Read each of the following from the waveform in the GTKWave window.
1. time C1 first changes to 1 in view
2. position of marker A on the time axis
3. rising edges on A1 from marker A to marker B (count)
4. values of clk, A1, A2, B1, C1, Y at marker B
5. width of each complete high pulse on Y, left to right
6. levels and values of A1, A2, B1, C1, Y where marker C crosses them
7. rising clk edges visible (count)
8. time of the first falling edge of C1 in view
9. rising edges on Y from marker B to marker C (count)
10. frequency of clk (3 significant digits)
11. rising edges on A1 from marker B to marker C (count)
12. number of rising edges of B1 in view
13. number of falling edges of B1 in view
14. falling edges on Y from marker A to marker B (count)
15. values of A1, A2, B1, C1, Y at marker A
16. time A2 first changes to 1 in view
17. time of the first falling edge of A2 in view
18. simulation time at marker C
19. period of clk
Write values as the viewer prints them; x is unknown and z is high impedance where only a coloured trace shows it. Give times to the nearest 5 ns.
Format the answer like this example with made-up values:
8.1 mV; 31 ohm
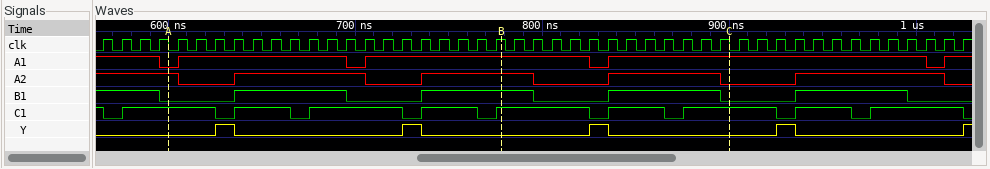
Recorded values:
575 ns; 600 ns; 2; clk=1, A1=1, A2=1, B1=1, C1=1, Y=0; 10 ns, 10 ns, 10 ns, 10 ns; A1=1, A2=0, B1=0, C1=1, Y=0; 47; 565 ns; 1; 100 MHz; 1; 4; 5; 2; A1=0, A2=1, B1=0, C1=1, Y=0; 635 ns; 605 ns; 900 ns; 10 ns
